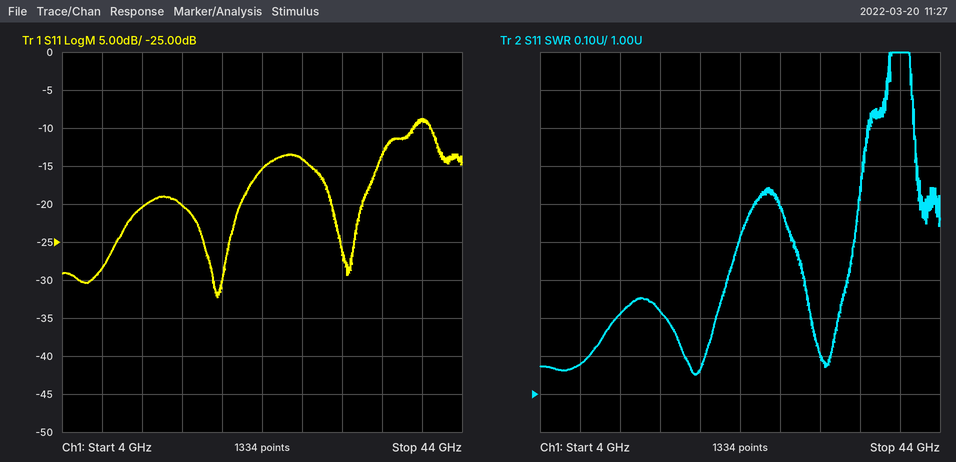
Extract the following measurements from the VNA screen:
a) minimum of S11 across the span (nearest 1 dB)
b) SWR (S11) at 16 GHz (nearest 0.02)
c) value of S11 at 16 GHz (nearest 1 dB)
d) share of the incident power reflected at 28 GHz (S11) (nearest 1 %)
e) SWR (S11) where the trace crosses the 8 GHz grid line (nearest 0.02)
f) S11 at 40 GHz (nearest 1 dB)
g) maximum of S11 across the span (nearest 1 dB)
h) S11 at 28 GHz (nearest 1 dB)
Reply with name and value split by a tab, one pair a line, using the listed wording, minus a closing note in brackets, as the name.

minimum of S11 across the span	-32 dB
SWR (S11) at 16 GHz	1.22
value of S11 at 16 GHz	-20 dB
share of the incident power reflected at 28 GHz (S11)	4 %
SWR (S11) where the trace crosses the 8 GHz grid line	1.08
S11 at 40 GHz	-9 dB
maximum of S11 across the span	-9 dB
S11 at 28 GHz	-14 dB
